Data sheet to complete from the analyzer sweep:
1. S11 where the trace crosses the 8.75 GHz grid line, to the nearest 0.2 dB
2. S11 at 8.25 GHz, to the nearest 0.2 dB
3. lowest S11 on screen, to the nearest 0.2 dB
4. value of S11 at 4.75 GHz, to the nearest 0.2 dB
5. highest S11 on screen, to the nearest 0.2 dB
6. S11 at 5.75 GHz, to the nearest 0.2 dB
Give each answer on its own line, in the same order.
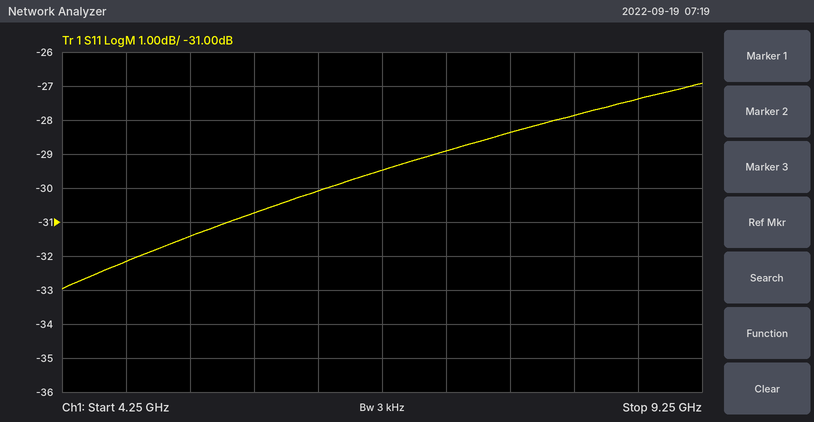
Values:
-27.4 dB
-27.8 dB
-33.0 dB
-32.2 dB
-27.0 dB
-30.8 dB
